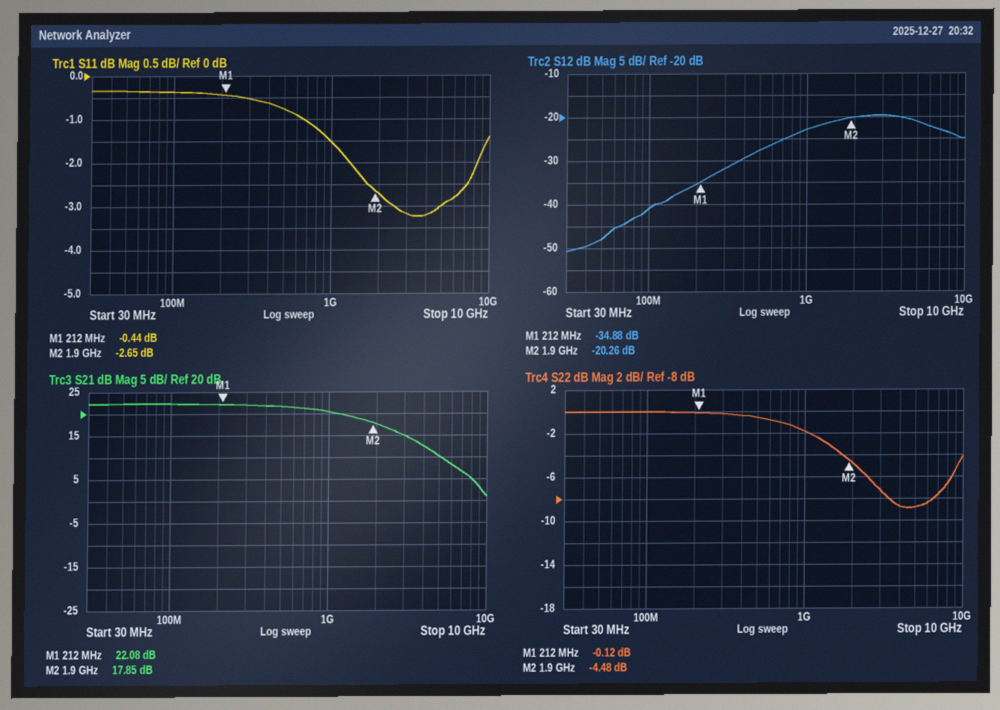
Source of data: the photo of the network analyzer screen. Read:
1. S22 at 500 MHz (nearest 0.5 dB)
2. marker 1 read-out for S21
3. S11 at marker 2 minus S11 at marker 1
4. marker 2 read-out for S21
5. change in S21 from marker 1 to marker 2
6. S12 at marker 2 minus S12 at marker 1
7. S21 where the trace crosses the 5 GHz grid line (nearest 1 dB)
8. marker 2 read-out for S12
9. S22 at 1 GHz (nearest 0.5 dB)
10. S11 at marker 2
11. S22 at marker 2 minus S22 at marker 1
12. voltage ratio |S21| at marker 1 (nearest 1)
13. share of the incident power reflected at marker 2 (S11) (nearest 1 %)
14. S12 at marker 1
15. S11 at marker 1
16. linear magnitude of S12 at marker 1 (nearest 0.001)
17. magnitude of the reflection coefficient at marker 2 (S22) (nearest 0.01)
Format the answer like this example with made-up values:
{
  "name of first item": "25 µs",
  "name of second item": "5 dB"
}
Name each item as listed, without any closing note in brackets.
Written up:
{
  "S22 at 500 MHz": "-0.5 dB",
  "marker 1 read-out for S21": "22.08 dB",
  "S11 at marker 2 minus S11 at marker 1": "-2.21 dB",
  "marker 2 read-out for S21": "17.85 dB",
  "change in S21 from marker 1 to marker 2": "-4.23 dB",
  "S12 at marker 2 minus S12 at marker 1": "14.62 dB",
  "S21 where the trace crosses the 5 GHz grid line": "10 dB",
  "marker 2 read-out for S12": "-20.26 dB",
  "S22 at 1 GHz": "-2.0 dB",
  "S11 at marker 2": "-2.65 dB",
  "S22 at marker 2 minus S22 at marker 1": "-4.36 dB",
  "voltage ratio |S21| at marker 1": "13",
  "share of the incident power reflected at marker 2 (S11)": "54 %",
  "S12 at marker 1": "-34.88 dB",
  "S11 at marker 1": "-0.44 dB",
  "linear magnitude of S12 at marker 1": "0.018",
  "magnitude of the reflection coefficient at marker 2 (S22)": "0.60"
}
